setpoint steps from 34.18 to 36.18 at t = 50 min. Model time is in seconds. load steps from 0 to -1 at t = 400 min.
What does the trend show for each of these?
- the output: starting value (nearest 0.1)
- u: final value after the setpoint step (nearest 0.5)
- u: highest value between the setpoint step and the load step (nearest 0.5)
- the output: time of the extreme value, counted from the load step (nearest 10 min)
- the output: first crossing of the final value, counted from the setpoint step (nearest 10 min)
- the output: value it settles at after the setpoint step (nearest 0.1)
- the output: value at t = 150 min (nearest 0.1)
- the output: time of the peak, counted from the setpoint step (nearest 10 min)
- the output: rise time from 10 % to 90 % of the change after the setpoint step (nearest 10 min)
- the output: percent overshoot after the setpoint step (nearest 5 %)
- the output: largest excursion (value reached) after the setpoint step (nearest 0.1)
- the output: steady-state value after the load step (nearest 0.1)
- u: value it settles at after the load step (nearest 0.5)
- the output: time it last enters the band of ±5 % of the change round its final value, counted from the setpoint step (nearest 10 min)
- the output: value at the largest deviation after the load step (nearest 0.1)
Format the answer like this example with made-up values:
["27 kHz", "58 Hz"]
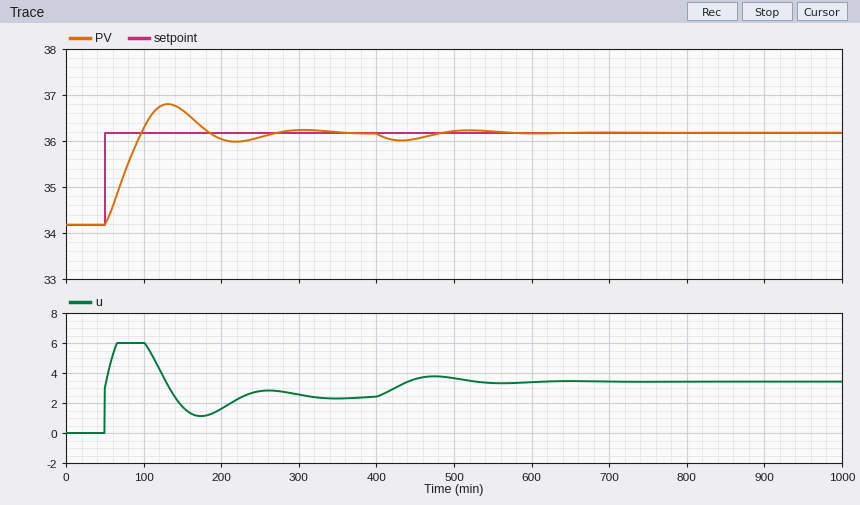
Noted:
["34.2", "2.5", "6.0", "30 min", "50 min", "36.2", "36.7", "80 min", "40 min", "30 %", "36.8", "36.2", "3.5", "200 min", "36.0"]
